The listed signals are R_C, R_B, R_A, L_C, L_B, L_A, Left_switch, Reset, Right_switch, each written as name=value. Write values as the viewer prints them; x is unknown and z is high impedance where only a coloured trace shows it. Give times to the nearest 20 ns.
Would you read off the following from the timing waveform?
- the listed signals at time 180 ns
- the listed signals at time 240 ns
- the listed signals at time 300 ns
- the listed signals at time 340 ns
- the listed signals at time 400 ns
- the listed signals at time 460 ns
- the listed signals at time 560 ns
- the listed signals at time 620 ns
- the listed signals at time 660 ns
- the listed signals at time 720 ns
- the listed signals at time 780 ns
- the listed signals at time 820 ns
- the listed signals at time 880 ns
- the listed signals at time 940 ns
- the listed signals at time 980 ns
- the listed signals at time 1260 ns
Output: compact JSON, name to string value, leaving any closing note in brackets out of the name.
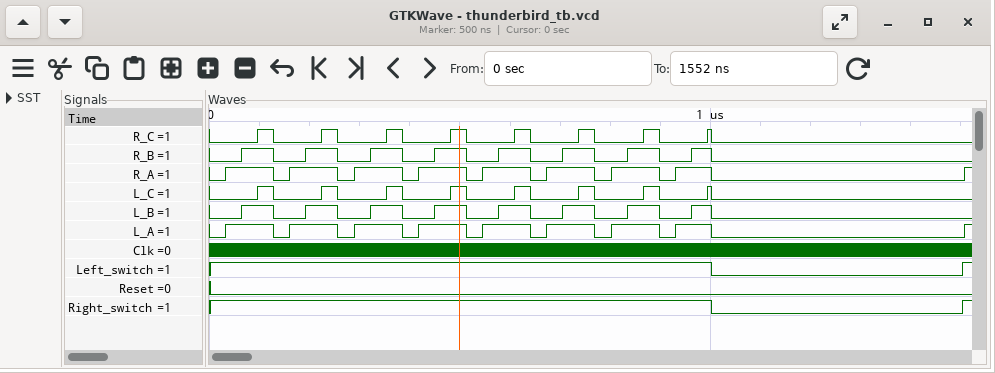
{"the listed signals at time 180 ns": "R_C=0, R_B=0, R_A=1, L_C=0, L_B=0, L_A=1, Left_switch=1, Reset=0, Right_switch=1", "the listed signals at time 240 ns": "R_C=1, R_B=1, R_A=1, L_C=1, L_B=1, L_A=1, Left_switch=1, Reset=0, Right_switch=1", "the listed signals at time 300 ns": "R_C=0, R_B=0, R_A=1, L_C=0, L_B=0, L_A=1, Left_switch=1, Reset=0, Right_switch=1", "the listed signals at time 340 ns": "R_C=0, R_B=1, R_A=1, L_C=0, L_B=1, L_A=1, Left_switch=1, Reset=0, Right_switch=1", "the listed signals at time 400 ns": "R_C=0, R_B=0, R_A=0, L_C=0, L_B=0, L_A=0, Left_switch=1, Reset=0, Right_switch=1", "the listed signals at time 460 ns": "R_C=0, R_B=1, R_A=1, L_C=0, L_B=1, L_A=1, Left_switch=1, Reset=0, Right_switch=1", "the listed signals at time 560 ns": "R_C=0, R_B=0, R_A=1, L_C=0, L_B=0, L_A=1, Left_switch=1, Reset=0, Right_switch=1", "the listed signals at time 620 ns": "R_C=1, R_B=1, R_A=1, L_C=1, L_B=1, L_A=1, Left_switch=1, Reset=0, Right_switch=1", "the listed signals at time 660 ns": "R_C=0, R_B=0, R_A=0, L_C=0, L_B=0, L_A=0, Left_switch=1, Reset=0, Right_switch=1", "the listed signals at time 720 ns": "R_C=0, R_B=1, R_A=1, L_C=0, L_B=1, L_A=1, Left_switch=1, Reset=0, Right_switch=1", "the listed signals at time 780 ns": "R_C=0, R_B=0, R_A=0, L_C=0, L_B=0, L_A=0, Left_switch=1, Reset=0, Right_switch=1", "the listed signals at time 820 ns": "R_C=0, R_B=0, R_A=1, L_C=0, L_B=0, L_A=1, Left_switch=1, Reset=0, Right_switch=1", "the listed signals at time 880 ns": "R_C=1, R_B=1, R_A=1, L_C=1, L_B=1, L_A=1, Left_switch=1, Reset=0, Right_switch=1", "the listed signals at time 940 ns": "R_C=0, R_B=0, R_A=1, L_C=0, L_B=0, L_A=1, Left_switch=1, Reset=0, Right_switch=1", "the listed signals at time 980 ns": "R_C=0, R_B=1, R_A=1, L_C=0, L_B=1, L_A=1, Left_switch=1, Reset=0, Right_switch=1", "the listed signals at time 1260 ns": "R_C=0, R_B=0, R_A=0, L_C=0, L_B=0, L_A=0, Left_switch=0, Reset=0, Right_switch=0"}
